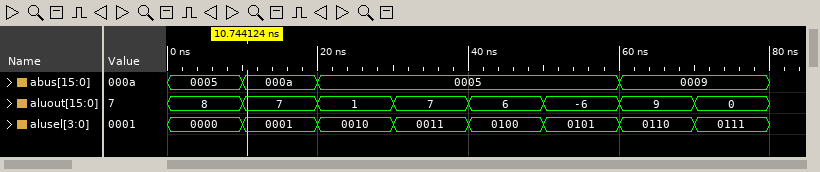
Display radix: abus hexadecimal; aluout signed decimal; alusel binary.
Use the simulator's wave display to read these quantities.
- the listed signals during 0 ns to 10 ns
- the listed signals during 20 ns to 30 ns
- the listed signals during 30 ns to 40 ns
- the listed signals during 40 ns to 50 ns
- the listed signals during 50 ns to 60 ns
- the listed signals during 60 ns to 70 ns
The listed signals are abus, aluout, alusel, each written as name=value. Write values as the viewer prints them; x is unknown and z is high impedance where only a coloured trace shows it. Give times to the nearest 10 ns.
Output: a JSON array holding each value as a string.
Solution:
["abus=0005, aluout=8, alusel=0000", "abus=0005, aluout=1, alusel=0010", "abus=0005, aluout=7, alusel=0011", "abus=0005, aluout=6, alusel=0100", "abus=0005, aluout=-6, alusel=0101", "abus=0009, aluout=9, alusel=0110"]
